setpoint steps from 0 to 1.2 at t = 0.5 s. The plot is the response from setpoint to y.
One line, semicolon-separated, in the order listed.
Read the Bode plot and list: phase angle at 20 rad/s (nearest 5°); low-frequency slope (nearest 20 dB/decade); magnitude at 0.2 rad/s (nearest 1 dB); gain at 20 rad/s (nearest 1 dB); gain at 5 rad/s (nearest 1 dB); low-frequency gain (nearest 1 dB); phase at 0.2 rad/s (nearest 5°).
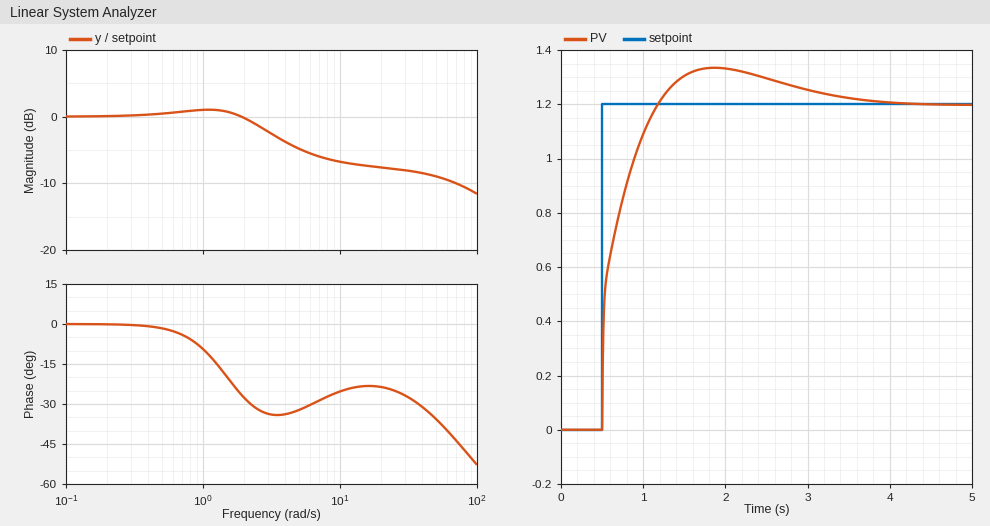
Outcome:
-25°; 0 dB/decade; 0 dB; -8 dB; -5 dB; 0 dB; 0°
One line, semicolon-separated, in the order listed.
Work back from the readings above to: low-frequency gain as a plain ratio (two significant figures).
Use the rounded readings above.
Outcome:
1.0
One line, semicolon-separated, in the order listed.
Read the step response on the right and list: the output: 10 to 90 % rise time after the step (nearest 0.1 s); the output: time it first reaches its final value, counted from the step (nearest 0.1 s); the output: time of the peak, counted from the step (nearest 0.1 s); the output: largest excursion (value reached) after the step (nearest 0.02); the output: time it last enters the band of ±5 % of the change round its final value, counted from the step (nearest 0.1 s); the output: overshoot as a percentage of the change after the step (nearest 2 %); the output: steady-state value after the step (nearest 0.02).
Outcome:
0.5 s; 0.7 s; 1.4 s; 1.34; 2.4 s; 12 %; 1.20
